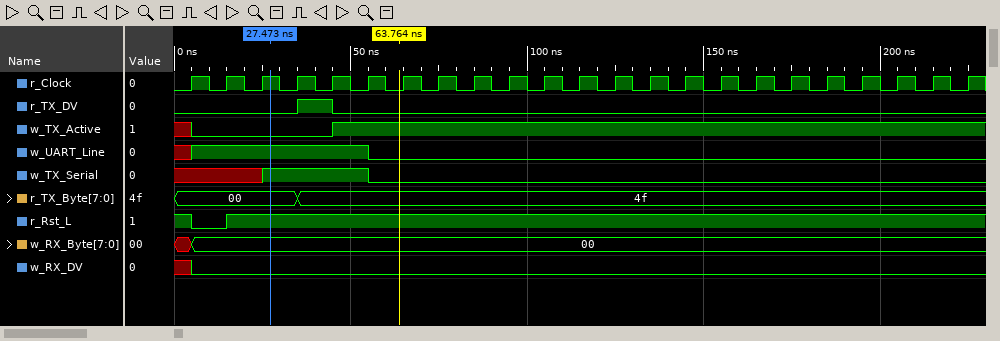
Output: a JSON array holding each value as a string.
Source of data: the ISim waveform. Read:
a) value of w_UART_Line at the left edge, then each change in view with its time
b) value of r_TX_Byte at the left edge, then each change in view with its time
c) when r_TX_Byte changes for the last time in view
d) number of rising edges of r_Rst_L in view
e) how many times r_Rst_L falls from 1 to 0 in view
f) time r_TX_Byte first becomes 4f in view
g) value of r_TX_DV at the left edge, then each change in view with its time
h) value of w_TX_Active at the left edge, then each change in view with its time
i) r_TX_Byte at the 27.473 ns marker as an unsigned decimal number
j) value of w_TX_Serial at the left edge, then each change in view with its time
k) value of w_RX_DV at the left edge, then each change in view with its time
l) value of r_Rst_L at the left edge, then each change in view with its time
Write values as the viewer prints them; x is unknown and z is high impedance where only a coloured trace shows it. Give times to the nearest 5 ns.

["x, 1 at 5 ns, 0 at 55 ns", "00, 4f at 35 ns", "35 ns", "1", "1", "35 ns", "0, 1 at 35 ns, 0 at 45 ns", "x, 0 at 5 ns, 1 at 45 ns", "0", "x, 1 at 25 ns, 0 at 55 ns", "x, 0 at 5 ns", "1, 0 at 5 ns, 1 at 15 ns"]
